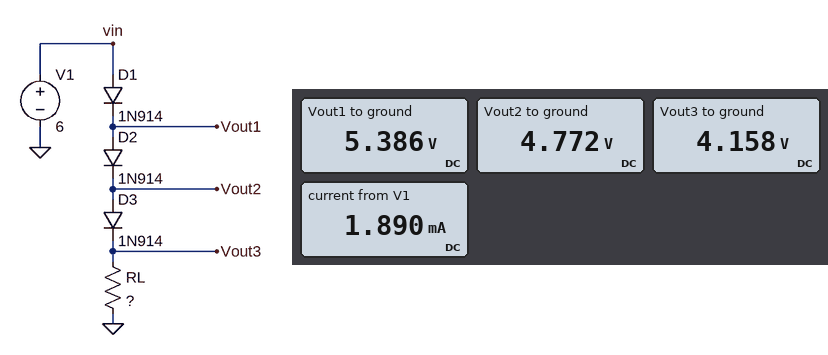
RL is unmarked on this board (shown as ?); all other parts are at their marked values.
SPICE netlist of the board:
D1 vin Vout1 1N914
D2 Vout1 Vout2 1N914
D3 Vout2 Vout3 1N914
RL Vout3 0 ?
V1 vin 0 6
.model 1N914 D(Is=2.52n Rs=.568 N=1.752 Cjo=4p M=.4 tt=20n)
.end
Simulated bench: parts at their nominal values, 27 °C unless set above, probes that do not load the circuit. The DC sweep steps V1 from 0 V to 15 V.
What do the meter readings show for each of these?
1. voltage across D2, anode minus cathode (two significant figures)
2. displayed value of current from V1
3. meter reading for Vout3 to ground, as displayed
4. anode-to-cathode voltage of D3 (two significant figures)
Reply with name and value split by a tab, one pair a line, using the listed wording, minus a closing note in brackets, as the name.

voltage across D2, anode minus cathode	610 mV
displayed value of current from V1	1.890 mA
meter reading for Vout3 to ground, as displayed	4.158 V
anode-to-cathode voltage of D3	610 mV
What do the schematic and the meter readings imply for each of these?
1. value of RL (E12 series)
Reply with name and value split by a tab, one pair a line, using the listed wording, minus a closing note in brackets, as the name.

value of RL	2.2 kΩ
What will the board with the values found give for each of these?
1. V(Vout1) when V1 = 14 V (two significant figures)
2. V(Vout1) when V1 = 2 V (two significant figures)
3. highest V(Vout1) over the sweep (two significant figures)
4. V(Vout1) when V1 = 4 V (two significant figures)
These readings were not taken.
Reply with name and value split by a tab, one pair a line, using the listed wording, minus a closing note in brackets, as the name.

V(Vout1) when V1 = 14 V	13 V
V(Vout1) when V1 = 2 V	1.5 V
highest V(Vout1) over the sweep	14 V
V(Vout1) when V1 = 4 V	3.4 V
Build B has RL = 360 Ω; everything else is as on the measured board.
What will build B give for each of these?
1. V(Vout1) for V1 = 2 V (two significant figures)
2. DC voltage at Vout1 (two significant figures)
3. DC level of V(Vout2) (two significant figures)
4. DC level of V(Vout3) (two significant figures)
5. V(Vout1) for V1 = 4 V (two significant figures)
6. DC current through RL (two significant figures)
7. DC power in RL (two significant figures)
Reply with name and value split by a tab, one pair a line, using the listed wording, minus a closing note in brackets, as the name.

V(Vout1) for V1 = 2 V	1.4 V
DC voltage at Vout1	5.3 V
DC level of V(Vout2)	4.6 V
DC level of V(Vout3)	3.9 V
V(Vout1) for V1 = 4 V	3.3 V
DC current through RL	11 mA
DC power in RL	42 mW
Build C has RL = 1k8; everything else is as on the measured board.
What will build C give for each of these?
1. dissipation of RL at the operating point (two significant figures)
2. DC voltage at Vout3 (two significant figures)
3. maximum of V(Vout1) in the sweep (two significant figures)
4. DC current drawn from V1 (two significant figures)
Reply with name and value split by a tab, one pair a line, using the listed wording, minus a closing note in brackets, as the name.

dissipation of RL at the operating point	9.5 mW
DC voltage at Vout3	4.1 V
maximum of V(Vout1) in the sweep	14 V
DC current drawn from V1	2.3 mA
